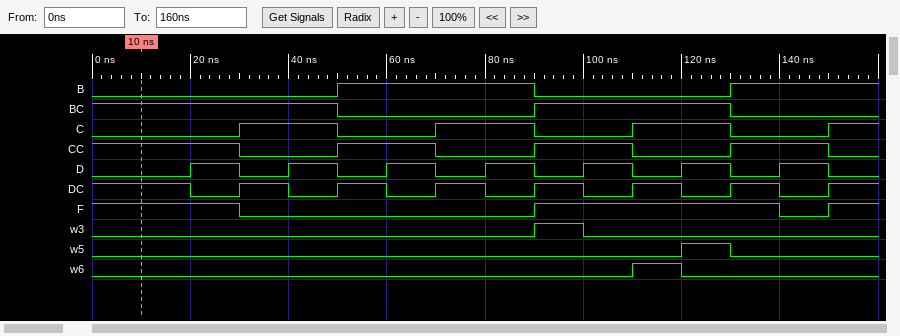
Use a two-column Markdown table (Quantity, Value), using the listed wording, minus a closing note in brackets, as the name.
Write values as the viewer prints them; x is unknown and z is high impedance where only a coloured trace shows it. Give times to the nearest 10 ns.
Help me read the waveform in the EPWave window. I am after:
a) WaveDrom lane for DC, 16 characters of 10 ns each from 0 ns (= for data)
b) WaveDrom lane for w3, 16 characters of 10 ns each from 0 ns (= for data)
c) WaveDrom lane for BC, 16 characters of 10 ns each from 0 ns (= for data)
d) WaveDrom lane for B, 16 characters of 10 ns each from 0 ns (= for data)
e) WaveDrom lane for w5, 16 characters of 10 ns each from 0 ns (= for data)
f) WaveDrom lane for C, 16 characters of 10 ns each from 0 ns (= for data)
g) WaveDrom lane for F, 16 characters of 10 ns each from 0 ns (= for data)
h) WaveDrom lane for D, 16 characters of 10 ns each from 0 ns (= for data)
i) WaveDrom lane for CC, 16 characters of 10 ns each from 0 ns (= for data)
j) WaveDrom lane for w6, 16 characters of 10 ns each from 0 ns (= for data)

| Quantity | Value |
|---|---|
| WaveDrom lane for DC, 16 characters of 10 ns each from 0 ns | {name: 'DC', wave: '1.01010101010101'} |
| WaveDrom lane for w3, 16 characters of 10 ns each from 0 ns | {name: 'w3', wave: '0........10.....'} |
| WaveDrom lane for BC, 16 characters of 10 ns each from 0 ns | {name: 'BC', wave: '1....0...1...0..'} |
| WaveDrom lane for B, 16 characters of 10 ns each from 0 ns | {name: 'B', wave: '0....1...0...1..'} |
| WaveDrom lane for w5, 16 characters of 10 ns each from 0 ns | {name: 'w5', wave: '0...........10..'} |
| WaveDrom lane for C, 16 characters of 10 ns each from 0 ns | {name: 'C', wave: '0..1.0.1.0.1.0.1'} |
| WaveDrom lane for F, 16 characters of 10 ns each from 0 ns | {name: 'F', wave: '1..0.....1....01'} |
| WaveDrom lane for D, 16 characters of 10 ns each from 0 ns | {name: 'D', wave: '0.10101010101010'} |
| WaveDrom lane for CC, 16 characters of 10 ns each from 0 ns | {name: 'CC', wave: '1..0.1.0.1.0.1.0'} |
| WaveDrom lane for w6, 16 characters of 10 ns each from 0 ns | {name: 'w6', wave: '0..........10...'} |
